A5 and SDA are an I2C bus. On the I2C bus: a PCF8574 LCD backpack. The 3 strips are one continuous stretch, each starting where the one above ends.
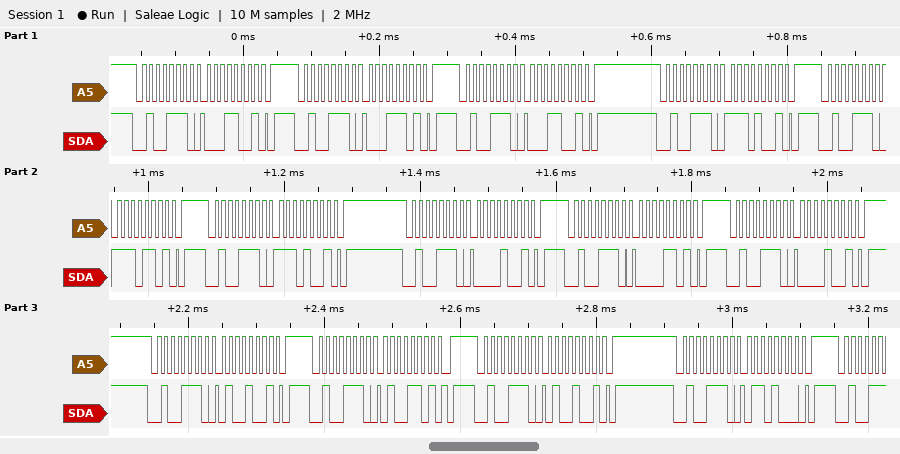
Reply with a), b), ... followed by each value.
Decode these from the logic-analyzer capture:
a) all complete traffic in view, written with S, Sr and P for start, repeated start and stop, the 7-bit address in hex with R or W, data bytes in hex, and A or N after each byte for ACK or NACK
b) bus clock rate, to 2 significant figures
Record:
a) S 27W A 19 A P S 27W A 1D A P S 27W A 19 A P S 27W A E9 A P S 27W A ED A P S 27W A E9 A P S 27W A 09 A P S 27W A 0D A P S 27W A 09 A P S 27W A 49 A P S 27W A 4D A P S 27W A 49 A P S 27W A 68 A P
b) 100 kHz
